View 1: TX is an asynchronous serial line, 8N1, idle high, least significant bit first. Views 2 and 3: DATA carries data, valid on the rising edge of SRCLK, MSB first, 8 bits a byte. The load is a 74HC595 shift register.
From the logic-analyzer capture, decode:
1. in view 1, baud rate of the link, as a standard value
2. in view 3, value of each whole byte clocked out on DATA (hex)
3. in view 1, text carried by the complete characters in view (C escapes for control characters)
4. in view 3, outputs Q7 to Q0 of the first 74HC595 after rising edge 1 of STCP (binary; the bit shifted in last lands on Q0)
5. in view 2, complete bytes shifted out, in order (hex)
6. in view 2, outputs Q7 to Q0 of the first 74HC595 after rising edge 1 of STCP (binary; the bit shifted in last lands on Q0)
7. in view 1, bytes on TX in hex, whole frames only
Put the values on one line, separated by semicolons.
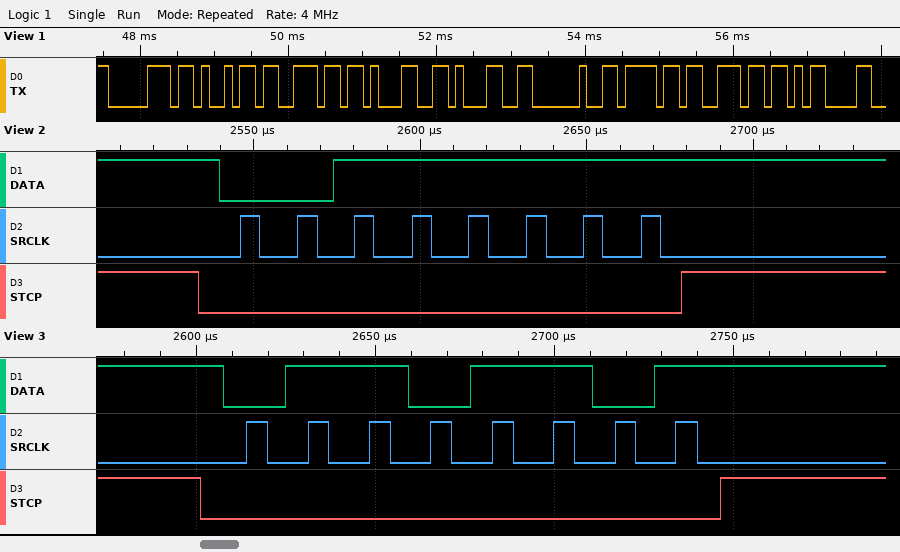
9600 baud; 6D; "pin11 on\r"; 01101101; 0x3F; 00111111; 70 69 6E 31 31 20 6F 6E 0D
